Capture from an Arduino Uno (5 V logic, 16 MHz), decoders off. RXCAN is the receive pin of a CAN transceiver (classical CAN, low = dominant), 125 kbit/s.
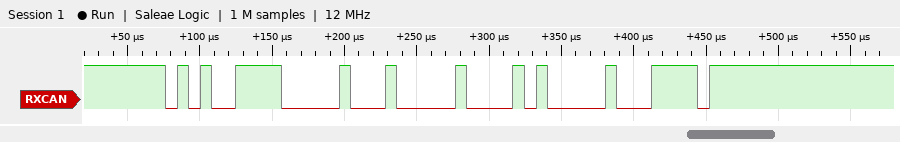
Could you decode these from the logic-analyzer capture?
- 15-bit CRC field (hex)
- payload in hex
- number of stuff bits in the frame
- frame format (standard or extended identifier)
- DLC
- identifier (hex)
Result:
0x2807
00
3
standard
1
0x53C
